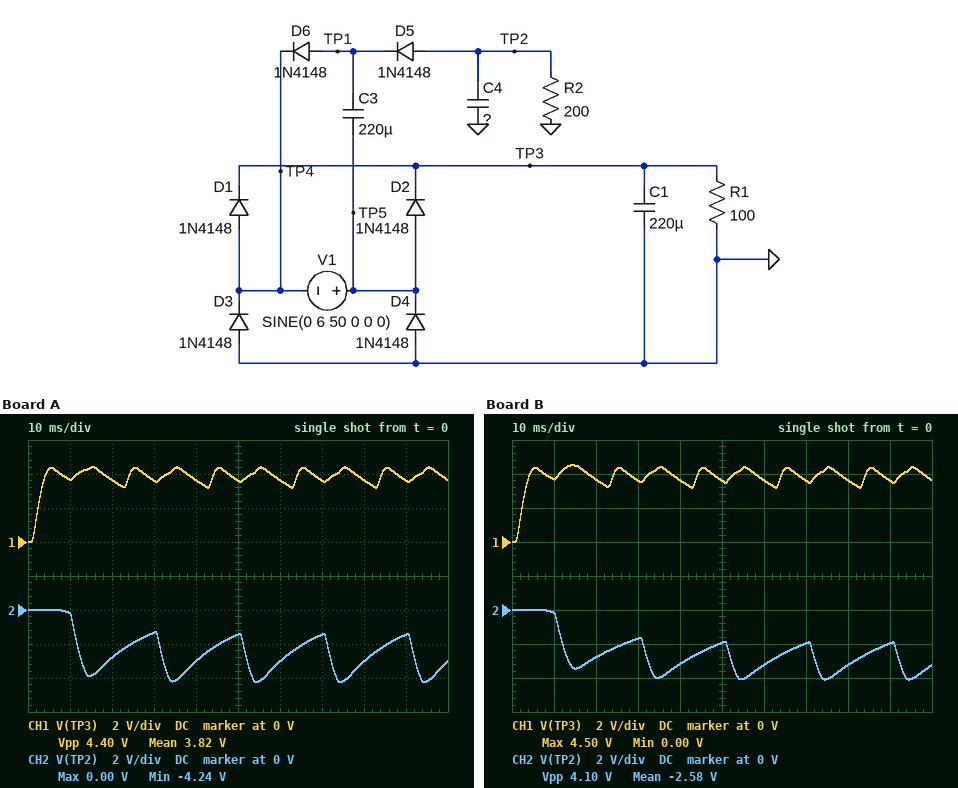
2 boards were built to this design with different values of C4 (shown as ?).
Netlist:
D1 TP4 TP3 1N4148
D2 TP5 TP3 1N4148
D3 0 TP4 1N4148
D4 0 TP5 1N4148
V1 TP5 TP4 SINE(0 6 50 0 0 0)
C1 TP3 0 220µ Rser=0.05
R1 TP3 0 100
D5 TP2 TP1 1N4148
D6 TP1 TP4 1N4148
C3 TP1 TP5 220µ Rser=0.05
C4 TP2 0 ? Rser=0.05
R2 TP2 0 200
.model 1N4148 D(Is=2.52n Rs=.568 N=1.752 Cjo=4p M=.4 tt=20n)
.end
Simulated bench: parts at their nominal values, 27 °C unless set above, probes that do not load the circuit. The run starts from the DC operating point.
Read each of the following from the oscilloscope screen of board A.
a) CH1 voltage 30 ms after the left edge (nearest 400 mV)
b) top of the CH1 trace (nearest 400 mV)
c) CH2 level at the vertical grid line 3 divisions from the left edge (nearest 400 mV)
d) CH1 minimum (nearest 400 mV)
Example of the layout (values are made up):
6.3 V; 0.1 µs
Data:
3.6 V; 4.4 V; -1.2 V; 0 V
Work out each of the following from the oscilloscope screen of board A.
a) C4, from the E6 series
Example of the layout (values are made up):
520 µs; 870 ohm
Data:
68 µF
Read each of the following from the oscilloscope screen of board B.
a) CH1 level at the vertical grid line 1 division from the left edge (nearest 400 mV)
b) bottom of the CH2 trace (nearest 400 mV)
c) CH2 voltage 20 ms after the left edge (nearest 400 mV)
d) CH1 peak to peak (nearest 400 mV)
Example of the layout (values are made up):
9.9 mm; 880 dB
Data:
3.6 V; -4.0 V; -2.8 V; 4.4 V
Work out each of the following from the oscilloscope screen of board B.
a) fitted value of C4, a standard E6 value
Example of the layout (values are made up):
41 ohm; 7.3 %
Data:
100 µF
